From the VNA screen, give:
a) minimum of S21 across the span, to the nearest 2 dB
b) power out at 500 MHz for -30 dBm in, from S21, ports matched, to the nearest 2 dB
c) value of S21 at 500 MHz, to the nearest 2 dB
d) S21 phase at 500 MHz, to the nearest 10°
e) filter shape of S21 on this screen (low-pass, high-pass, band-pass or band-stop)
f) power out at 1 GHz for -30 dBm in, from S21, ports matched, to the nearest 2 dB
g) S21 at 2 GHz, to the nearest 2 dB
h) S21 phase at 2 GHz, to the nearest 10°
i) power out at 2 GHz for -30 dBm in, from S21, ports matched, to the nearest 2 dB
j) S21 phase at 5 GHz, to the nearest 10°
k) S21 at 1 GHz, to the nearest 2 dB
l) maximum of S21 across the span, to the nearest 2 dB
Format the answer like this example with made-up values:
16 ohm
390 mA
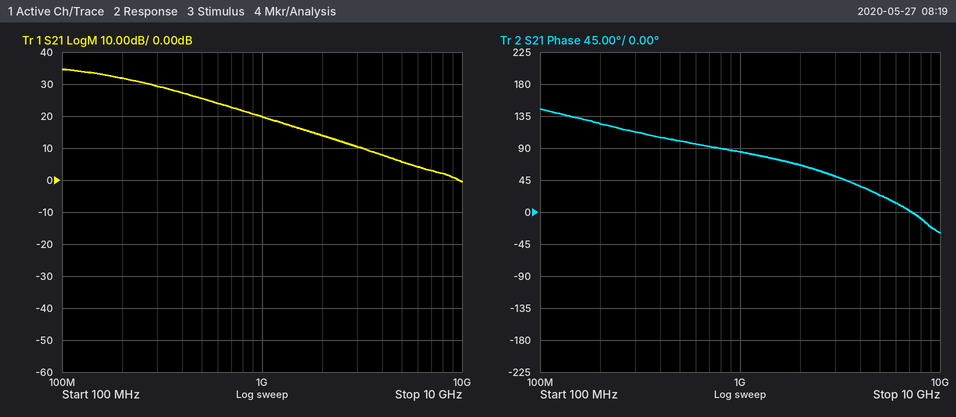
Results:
0 dB
-4 dBm
26 dB
100°
low-pass
-10 dBm
14 dB
70°
-16 dBm
20°
20 dB
34 dB
